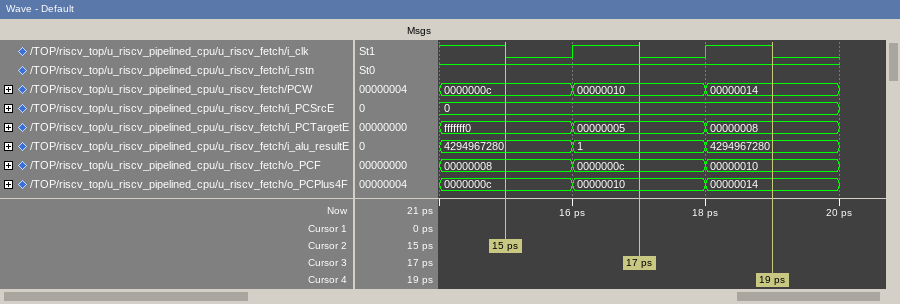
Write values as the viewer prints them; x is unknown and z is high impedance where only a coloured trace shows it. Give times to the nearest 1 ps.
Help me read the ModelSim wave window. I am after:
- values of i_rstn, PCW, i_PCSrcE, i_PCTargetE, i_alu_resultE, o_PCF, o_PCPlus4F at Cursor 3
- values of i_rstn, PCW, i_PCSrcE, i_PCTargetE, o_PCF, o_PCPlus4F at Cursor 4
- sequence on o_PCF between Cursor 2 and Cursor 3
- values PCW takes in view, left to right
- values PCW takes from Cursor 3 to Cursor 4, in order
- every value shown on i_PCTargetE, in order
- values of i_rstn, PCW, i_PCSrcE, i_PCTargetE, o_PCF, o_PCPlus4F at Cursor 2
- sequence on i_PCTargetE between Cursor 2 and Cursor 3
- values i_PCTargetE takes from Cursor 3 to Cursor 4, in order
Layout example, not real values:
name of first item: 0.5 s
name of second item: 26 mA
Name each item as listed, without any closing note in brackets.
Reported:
values of i_rstn, PCW, i_PCSrcE, i_PCTargetE, i_alu_resultE, o_PCF, o_PCPlus4F at Cursor 3: i_rstn=1, PCW=00000010, i_PCSrcE=0, i_PCTargetE=00000005, i_alu_resultE=1, o_PCF=0000000c, o_PCPlus4F=00000010
values of i_rstn, PCW, i_PCSrcE, i_PCTargetE, o_PCF, o_PCPlus4F at Cursor 4: i_rstn=1, PCW=00000014, i_PCSrcE=0, i_PCTargetE=00000008, o_PCF=00000010, o_PCPlus4F=00000014
sequence on o_PCF between Cursor 2 and Cursor 3: 00000008, 0000000c
values PCW takes in view, left to right: 0000000c, 00000010, 00000014
values PCW takes from Cursor 3 to Cursor 4, in order: 00000010, 00000014
every value shown on i_PCTargetE, in order: fffffff0, 00000005, 00000008
values of i_rstn, PCW, i_PCSrcE, i_PCTargetE, o_PCF, o_PCPlus4F at Cursor 2: i_rstn=1, PCW=0000000c, i_PCSrcE=0, i_PCTargetE=fffffff0, o_PCF=00000008, o_PCPlus4F=0000000c
sequence on i_PCTargetE between Cursor 2 and Cursor 3: fffffff0, 00000005
values i_PCTargetE takes from Cursor 3 to Cursor 4, in order: 00000005, 00000008
